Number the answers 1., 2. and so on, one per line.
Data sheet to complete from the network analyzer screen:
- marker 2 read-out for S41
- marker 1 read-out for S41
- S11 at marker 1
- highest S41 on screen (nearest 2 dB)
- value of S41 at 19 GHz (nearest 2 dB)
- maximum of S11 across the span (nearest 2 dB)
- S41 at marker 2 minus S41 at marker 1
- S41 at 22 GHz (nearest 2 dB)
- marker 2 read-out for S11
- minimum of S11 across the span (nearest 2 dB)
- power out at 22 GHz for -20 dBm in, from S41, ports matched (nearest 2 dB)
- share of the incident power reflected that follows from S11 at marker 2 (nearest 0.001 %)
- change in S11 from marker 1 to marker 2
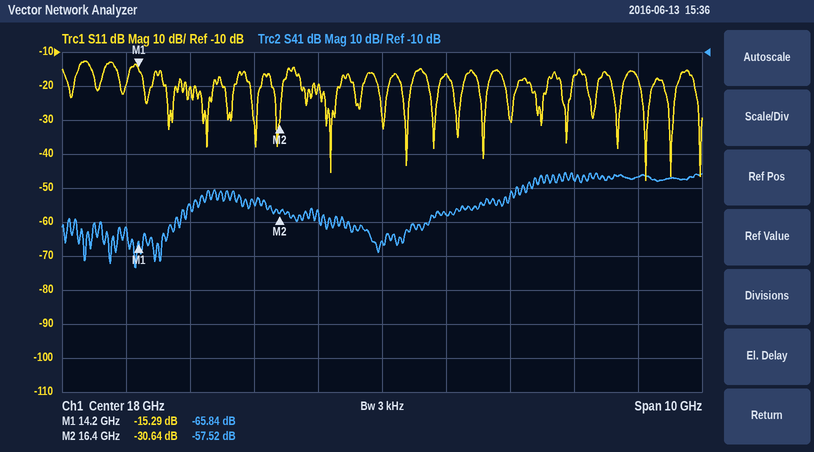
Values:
1. -57.52 dB
2. -65.84 dB
3. -15.29 dB
4. -46 dB
5. -58 dB
6. -12 dB
7. 8.32 dB
8. -46 dB
9. -30.64 dB
10. -48 dB
11. -66 dBm
12. 0.086 %
13. -15.35 dB
